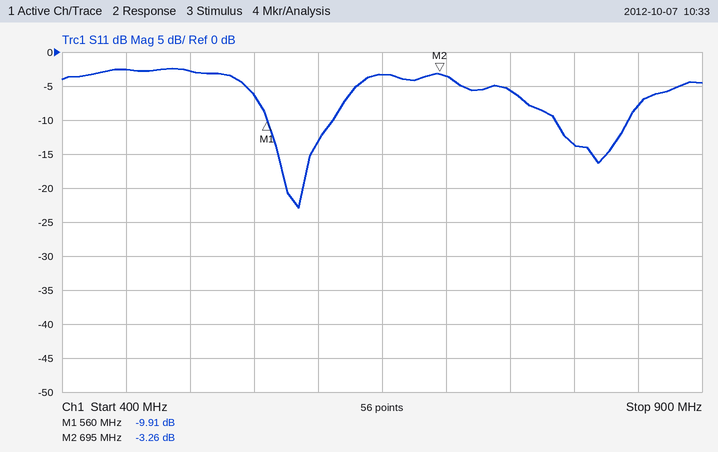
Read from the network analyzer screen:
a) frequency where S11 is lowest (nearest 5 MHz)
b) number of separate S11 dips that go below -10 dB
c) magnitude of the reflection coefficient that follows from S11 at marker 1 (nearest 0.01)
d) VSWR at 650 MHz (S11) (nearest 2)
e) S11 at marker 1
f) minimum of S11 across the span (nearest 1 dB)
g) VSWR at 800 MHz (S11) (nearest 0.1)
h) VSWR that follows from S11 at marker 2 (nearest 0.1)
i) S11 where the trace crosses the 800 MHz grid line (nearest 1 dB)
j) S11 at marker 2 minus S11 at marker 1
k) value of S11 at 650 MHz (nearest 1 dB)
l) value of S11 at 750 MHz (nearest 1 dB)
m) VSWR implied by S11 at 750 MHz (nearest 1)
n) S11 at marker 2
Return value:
585 MHz
2
0.32
6
-9.91 dB
-23 dB
1.5
5.4
-14 dB
6.65 dB
-3 dB
-6 dB
3
-3.26 dB
